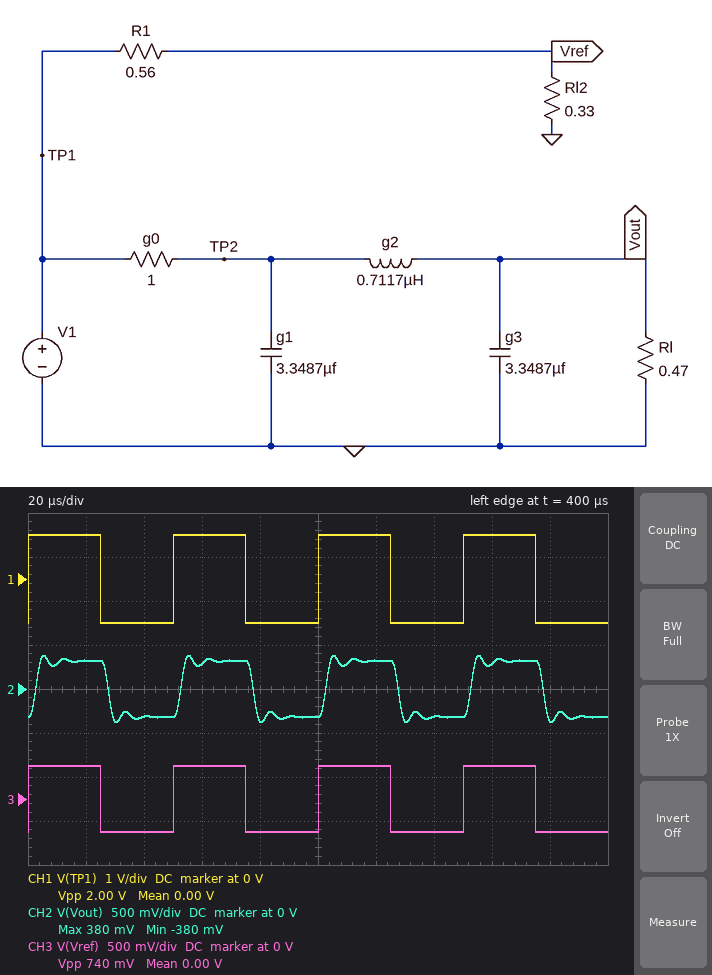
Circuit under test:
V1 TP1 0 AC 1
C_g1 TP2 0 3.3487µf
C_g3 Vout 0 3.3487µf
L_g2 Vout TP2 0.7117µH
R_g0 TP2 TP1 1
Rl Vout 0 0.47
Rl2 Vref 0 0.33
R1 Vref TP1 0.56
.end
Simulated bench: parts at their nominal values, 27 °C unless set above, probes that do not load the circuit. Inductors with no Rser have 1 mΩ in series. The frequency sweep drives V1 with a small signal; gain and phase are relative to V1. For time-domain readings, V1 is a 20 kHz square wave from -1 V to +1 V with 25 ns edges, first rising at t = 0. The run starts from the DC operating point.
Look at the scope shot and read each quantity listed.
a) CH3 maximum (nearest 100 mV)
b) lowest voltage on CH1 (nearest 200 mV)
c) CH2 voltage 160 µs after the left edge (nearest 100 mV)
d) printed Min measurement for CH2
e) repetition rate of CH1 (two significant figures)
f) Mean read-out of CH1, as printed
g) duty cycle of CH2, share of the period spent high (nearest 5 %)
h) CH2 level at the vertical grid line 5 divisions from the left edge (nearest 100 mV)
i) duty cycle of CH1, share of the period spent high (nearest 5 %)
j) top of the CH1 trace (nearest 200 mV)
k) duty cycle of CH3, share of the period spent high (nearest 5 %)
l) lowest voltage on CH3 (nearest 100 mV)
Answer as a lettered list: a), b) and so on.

a) 400 mV
b) -1.0 V
c) 300 mV
d) -380 mV
e) 20 kHz
f) 0.00 V
g) 50 %
h) -300 mV
i) 50 %
j) 1.0 V
k) 50 %
l) -400 mV
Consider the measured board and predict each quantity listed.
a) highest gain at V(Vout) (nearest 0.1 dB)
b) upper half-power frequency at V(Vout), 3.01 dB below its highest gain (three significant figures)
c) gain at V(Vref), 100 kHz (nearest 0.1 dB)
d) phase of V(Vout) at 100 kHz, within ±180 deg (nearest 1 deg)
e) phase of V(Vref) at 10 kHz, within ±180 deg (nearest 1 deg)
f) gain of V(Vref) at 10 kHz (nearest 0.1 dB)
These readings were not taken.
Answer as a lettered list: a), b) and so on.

a) -9.5 dB
b) 158 kHz
c) -8.6 dB
d) -87 deg
e) 0 deg
f) -8.6 dB
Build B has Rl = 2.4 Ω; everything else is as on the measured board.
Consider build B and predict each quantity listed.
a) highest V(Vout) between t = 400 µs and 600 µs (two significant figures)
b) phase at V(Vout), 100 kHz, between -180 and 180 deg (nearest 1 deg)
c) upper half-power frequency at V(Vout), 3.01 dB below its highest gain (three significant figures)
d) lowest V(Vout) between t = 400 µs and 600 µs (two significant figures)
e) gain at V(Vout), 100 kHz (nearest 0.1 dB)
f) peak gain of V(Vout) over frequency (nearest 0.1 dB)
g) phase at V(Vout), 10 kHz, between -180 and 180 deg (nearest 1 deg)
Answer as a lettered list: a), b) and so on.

a) 730 mV
b) -88 deg
c) 156 kHz
d) -730 mV
e) -7.7 dB
f) -2.9 dB
g) -17 deg
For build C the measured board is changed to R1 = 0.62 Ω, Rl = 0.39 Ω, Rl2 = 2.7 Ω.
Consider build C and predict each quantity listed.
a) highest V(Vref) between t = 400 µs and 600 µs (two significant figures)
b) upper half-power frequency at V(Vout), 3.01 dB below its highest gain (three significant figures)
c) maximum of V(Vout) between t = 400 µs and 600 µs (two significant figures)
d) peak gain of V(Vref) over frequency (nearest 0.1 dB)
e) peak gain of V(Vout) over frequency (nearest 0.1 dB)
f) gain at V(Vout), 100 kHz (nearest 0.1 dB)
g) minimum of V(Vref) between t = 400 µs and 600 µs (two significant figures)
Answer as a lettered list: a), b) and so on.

a) 810 mV
b) 155 kHz
c) 350 mV
d) -1.8 dB
e) -10.3 dB
f) -10.6 dB
g) -810 mV
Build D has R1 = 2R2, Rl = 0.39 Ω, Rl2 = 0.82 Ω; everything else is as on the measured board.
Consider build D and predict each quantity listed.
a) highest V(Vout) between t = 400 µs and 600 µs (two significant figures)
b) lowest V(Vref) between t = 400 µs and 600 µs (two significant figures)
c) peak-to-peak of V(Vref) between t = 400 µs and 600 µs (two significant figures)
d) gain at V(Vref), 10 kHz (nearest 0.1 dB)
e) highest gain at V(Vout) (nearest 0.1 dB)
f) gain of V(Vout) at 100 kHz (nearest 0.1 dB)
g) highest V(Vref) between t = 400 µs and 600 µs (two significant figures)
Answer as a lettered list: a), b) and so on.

a) 350 mV
b) -270 mV
c) 540 mV
d) -11.3 dB
e) -10.3 dB
f) -10.6 dB
g) 270 mV
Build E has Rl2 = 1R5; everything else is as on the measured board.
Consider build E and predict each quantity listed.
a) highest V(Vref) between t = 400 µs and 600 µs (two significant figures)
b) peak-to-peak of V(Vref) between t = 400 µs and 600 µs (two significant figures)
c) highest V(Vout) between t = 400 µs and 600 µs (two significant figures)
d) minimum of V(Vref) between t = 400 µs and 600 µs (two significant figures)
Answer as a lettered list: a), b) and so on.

a) 730 mV
b) 1.5 V
c) 380 mV
d) -730 mV
